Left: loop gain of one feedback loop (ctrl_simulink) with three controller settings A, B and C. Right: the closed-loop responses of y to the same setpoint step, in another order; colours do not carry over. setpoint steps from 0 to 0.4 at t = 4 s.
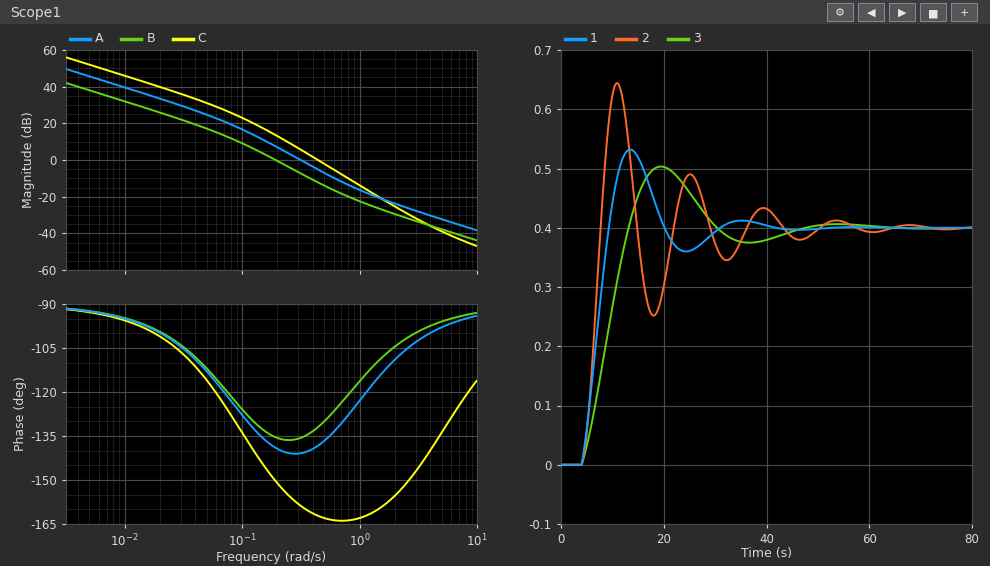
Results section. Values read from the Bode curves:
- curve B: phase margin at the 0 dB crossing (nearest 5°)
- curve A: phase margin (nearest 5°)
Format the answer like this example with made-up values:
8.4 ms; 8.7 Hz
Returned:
45°; 40°
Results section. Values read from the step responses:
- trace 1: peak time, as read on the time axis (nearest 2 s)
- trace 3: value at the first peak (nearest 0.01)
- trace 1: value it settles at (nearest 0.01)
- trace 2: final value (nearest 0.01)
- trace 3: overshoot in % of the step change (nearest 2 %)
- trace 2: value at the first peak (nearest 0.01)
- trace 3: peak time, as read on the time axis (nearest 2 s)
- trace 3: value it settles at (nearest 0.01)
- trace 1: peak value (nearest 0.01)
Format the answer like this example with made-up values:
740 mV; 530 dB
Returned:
14 s; 0.50; 0.40; 0.40; 26 %; 0.64; 20 s; 0.40; 0.53
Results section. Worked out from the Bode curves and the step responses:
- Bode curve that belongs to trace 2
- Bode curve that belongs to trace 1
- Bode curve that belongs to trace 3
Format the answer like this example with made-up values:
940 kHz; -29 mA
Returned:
C; A; B
